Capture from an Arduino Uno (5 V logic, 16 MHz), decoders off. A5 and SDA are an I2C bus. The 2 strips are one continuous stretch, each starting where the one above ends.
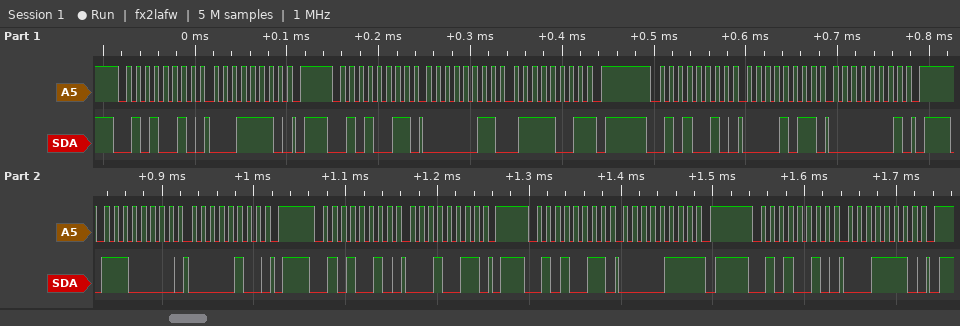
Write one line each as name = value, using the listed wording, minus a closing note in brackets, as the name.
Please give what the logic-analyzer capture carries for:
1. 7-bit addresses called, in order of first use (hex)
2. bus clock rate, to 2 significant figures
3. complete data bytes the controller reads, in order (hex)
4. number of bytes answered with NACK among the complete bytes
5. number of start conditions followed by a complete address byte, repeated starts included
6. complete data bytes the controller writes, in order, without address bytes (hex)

7-bit addresses called, in order of first use = 0x29 0x70
bus clock rate, to 2 significant figures = 100 kHz
complete data bytes the controller reads, in order = 03 79 07
number of bytes answered with NACK among the complete bytes = 2
number of start conditions followed by a complete address byte, repeated starts included = 7
complete data bytes the controller writes, in order, without address bytes = 1E 0B 01 04 13 1E
